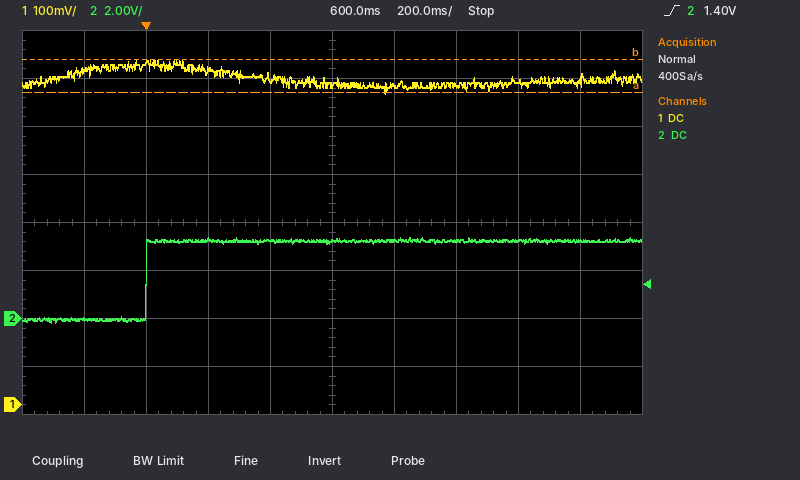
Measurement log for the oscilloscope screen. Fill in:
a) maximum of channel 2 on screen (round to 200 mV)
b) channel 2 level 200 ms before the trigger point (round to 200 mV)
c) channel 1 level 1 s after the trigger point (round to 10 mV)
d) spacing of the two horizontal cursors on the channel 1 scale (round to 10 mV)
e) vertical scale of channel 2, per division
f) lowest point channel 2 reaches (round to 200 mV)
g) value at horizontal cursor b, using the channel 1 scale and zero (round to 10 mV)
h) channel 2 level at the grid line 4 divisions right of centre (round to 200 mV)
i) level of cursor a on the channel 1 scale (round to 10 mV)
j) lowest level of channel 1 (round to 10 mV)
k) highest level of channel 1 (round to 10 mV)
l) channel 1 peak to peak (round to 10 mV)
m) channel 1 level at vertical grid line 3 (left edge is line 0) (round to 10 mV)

3.4 V
0.0 V
670 mV
70 mV
2 V
-200 mV
720 mV
3.2 V
650 mV
650 mV
720 mV
70 mV
700 mV
